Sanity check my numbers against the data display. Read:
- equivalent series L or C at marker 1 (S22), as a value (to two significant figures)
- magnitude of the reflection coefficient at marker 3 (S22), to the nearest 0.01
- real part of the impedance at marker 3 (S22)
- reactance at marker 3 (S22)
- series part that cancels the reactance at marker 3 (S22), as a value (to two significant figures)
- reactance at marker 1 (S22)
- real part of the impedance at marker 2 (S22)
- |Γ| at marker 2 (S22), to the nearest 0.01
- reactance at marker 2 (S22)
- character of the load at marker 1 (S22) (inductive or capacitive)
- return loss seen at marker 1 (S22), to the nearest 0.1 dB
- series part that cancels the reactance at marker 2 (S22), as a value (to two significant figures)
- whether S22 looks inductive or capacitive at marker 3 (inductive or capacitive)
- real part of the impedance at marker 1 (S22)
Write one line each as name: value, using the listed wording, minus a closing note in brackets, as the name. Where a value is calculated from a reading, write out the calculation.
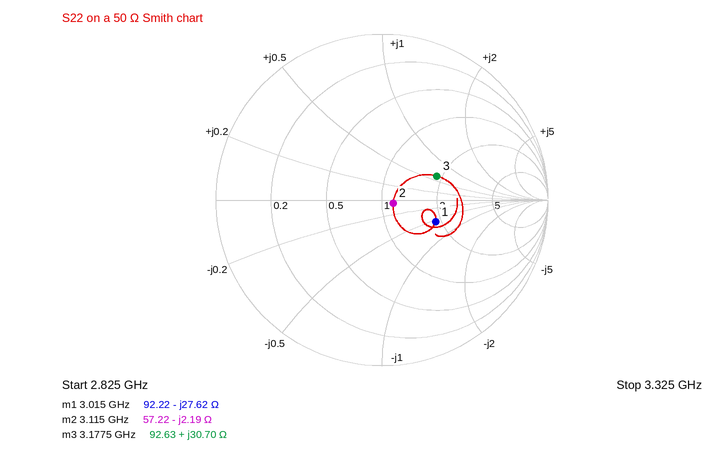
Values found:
equivalent series L or C at marker 1 (S22), as a value: C = 1/(2π × 3.015 GHz × 27.62 Ω) ≈ 1.9 pF
magnitude of the reflection coefficient at marker 3 (S22), to the nearest 0.01: 0.36
real part of the impedance at marker 3: 92.63 Ω
reactance at marker 3: +30.70 Ω
series part that cancels the reactance at marker 3 (S22), as a value: C = 1/(2π × 3.1775 GHz × 30.7 Ω) ≈ 1.6 pF
reactance at marker 1: -27.62 Ω
real part of the impedance at marker 2: 57.22 Ω
|Γ| at marker 2 (S22), to the nearest 0.01: 0.07
reactance at marker 2: -2.19 Ω
character of the load at marker 1 (S22): capacitive
return loss seen at marker 1 (S22), to the nearest 0.1 dB: 9.2 dB
series part that cancels the reactance at marker 2 (S22), as a value: L = 2.19 Ω/(2π × 3.115 GHz) ≈ 112 pH, so 110 pH to two significant figures
whether S22 looks inductive or capacitive at marker 3: inductive
real part of the impedance at marker 1: 92.22 Ω
